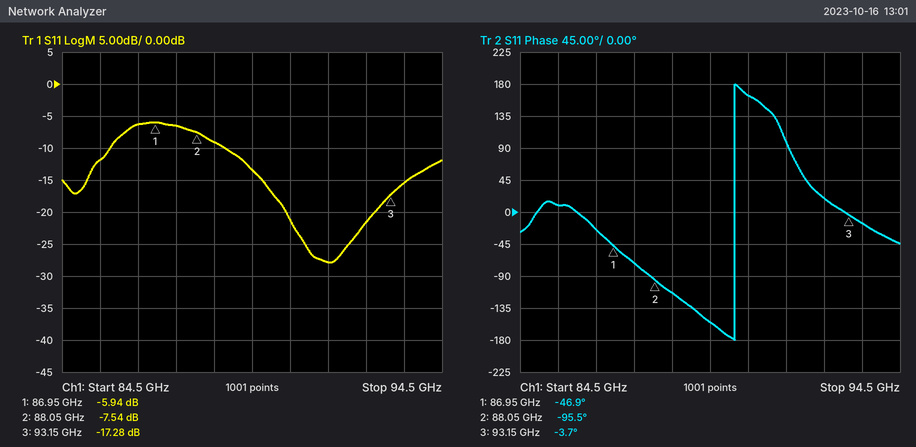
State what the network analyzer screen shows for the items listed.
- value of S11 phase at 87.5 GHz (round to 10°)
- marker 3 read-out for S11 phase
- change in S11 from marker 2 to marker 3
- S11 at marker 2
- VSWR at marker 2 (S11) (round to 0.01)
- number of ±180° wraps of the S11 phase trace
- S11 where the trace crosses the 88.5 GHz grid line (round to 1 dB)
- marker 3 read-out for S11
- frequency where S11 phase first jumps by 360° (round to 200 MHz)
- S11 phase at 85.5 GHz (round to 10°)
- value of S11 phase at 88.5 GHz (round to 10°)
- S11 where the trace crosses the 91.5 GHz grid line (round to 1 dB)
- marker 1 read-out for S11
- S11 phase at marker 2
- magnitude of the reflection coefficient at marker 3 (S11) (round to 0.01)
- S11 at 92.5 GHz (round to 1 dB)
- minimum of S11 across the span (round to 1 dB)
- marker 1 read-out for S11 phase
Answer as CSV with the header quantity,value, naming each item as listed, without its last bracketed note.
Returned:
quantity,value
value of S11 phase at 87.5 GHz,-70°
marker 3 read-out for S11 phase,-3.7°
change in S11 from marker 2 to marker 3,-9.74 dB
S11 at marker 2,-7.54 dB
VSWR at marker 2 (S11),2.45
number of ±180° wraps of the S11 phase trace,1
S11 where the trace crosses the 88.5 GHz grid line,-9 dB
marker 3 read-out for S11,-17.28 dB
frequency where S11 phase first jumps by 360°,90.2 GHz
S11 phase at 85.5 GHz,10°
value of S11 phase at 88.5 GHz,-110°
S11 where the trace crosses the 91.5 GHz grid line,-28 dB
marker 1 read-out for S11,-5.94 dB
S11 phase at marker 2,-95.5°
magnitude of the reflection coefficient at marker 3 (S11),0.14
S11 at 92.5 GHz,-22 dB
minimum of S11 across the span,-28 dB
marker 1 read-out for S11 phase,-46.9°
